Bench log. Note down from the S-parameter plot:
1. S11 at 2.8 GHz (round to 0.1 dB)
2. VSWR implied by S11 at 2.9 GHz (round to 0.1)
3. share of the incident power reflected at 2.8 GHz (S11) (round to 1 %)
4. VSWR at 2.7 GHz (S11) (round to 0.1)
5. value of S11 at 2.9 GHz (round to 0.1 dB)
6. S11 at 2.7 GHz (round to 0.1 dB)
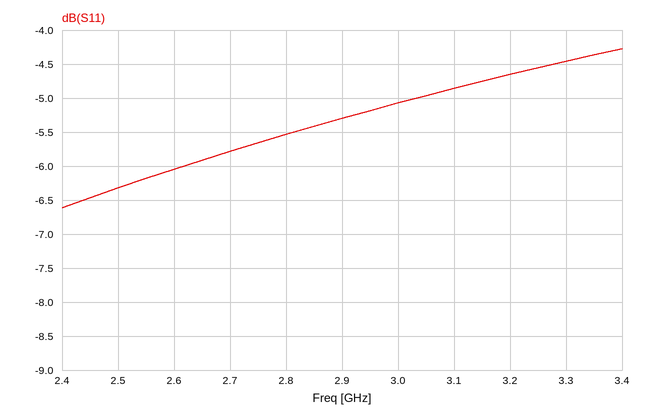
-5.5 dB
3.4
28 %
3.1
-5.3 dB
-5.8 dB
